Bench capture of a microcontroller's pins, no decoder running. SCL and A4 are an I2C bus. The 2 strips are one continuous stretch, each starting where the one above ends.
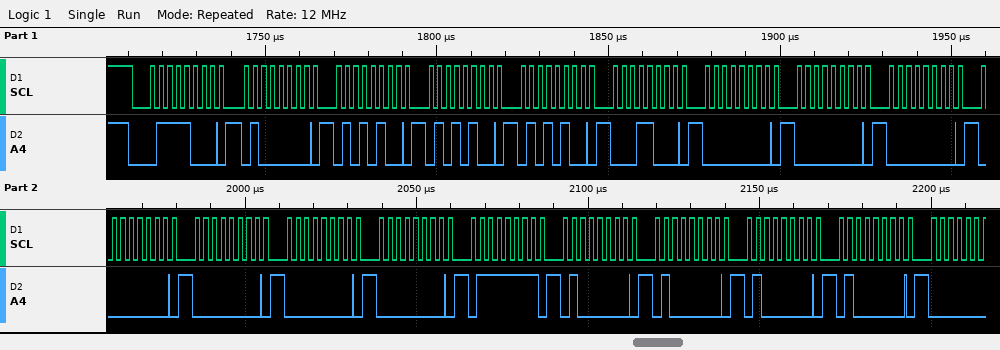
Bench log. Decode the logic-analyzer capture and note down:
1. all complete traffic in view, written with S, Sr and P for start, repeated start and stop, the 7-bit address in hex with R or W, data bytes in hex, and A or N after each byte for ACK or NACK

S 3CW A 40 A 54 A 54 A 54 A 18 A 00 A 00 A 00 A 00 A 00 A 00 A 00 A 7F A 40 A 40 A 40 A 40 A
